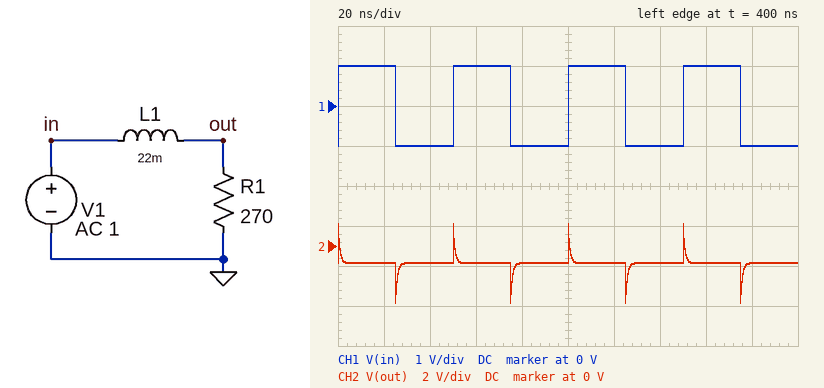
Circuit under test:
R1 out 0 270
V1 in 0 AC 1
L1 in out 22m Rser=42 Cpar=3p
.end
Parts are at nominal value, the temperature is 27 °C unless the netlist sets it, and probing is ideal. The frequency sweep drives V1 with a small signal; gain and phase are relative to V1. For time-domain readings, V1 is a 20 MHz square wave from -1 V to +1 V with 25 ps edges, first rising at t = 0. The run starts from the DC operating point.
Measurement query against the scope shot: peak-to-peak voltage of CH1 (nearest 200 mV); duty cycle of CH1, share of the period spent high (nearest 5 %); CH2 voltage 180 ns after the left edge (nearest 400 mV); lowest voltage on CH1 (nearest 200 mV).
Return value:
2.0 V
50 %
-800 mV
-1.0 V
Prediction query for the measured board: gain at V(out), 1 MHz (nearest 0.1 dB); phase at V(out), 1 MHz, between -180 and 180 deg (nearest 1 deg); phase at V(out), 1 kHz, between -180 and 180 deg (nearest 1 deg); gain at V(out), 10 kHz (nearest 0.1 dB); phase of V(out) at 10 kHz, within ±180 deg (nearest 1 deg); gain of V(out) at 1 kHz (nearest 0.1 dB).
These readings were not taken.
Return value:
-50.1 dB
90 deg
-24 deg
-14.4 dB
-77 deg
-2.0 dB
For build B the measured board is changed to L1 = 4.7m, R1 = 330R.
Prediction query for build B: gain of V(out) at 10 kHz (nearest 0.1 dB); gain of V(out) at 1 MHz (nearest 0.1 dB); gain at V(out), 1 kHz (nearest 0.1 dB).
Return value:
-3.2 dB
-46.1 dB
-1.1 dB
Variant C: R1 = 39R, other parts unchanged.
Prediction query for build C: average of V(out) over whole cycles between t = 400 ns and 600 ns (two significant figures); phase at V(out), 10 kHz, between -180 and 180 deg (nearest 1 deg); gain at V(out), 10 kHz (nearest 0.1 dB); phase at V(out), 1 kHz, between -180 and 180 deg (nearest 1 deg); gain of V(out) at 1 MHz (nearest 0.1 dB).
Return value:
-480 mV
-87 deg
-31.0 dB
-60 deg
-66.9 dB
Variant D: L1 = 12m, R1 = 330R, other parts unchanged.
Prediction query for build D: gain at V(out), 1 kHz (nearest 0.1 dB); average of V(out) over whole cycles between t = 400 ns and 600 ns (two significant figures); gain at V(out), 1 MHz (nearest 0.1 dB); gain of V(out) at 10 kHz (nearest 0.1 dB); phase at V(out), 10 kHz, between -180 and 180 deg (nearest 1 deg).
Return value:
-1.2 dB
-870 mV
-54.7 dB
-8.1 dB
-64 deg
